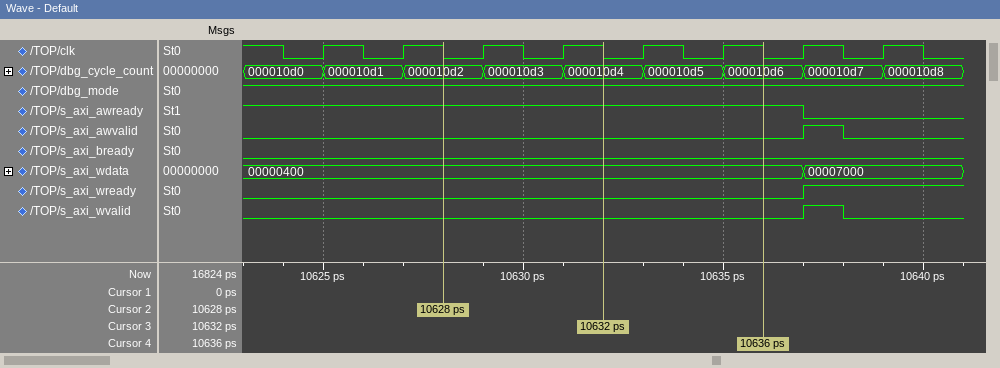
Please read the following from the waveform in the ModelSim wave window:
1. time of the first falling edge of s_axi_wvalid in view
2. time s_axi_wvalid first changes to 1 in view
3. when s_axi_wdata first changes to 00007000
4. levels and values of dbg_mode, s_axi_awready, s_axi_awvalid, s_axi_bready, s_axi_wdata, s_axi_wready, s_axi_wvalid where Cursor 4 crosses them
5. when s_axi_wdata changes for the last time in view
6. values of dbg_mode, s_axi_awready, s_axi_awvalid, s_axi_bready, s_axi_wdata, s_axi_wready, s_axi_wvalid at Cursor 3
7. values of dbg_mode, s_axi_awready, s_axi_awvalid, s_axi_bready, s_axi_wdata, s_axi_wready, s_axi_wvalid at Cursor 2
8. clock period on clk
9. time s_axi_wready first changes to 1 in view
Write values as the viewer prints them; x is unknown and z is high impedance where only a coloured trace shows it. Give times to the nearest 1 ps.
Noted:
10638 ps
10637 ps
10637 ps
dbg_mode=1, s_axi_awready=1, s_axi_awvalid=0, s_axi_bready=0, s_axi_wdata=00000400, s_axi_wready=0, s_axi_wvalid=0
10637 ps
dbg_mode=1, s_axi_awready=1, s_axi_awvalid=0, s_axi_bready=0, s_axi_wdata=00000400, s_axi_wready=0, s_axi_wvalid=0
dbg_mode=1, s_axi_awready=1, s_axi_awvalid=0, s_axi_bready=0, s_axi_wdata=00000400, s_axi_wready=0, s_axi_wvalid=0
2 ps
10637 ps
